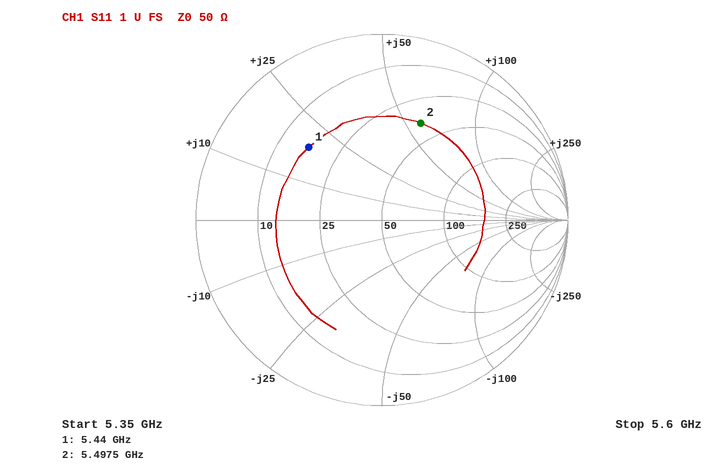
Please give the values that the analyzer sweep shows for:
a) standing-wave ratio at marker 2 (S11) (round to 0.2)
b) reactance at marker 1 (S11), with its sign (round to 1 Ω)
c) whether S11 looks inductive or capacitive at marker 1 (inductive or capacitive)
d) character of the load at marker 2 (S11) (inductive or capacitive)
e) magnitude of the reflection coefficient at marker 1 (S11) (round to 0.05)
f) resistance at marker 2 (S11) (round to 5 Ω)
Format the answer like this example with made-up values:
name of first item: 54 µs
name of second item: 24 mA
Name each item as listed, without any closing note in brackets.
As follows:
standing-wave ratio at marker 2 (S11): 3.6
reactance at marker 1 (S11), with its sign: +19 Ω
whether S11 looks inductive or capacitive at marker 1: inductive
character of the load at marker 2 (S11): inductive
magnitude of the reflection coefficient at marker 1 (S11): 0.55
resistance at marker 2 (S11): 40 Ω
